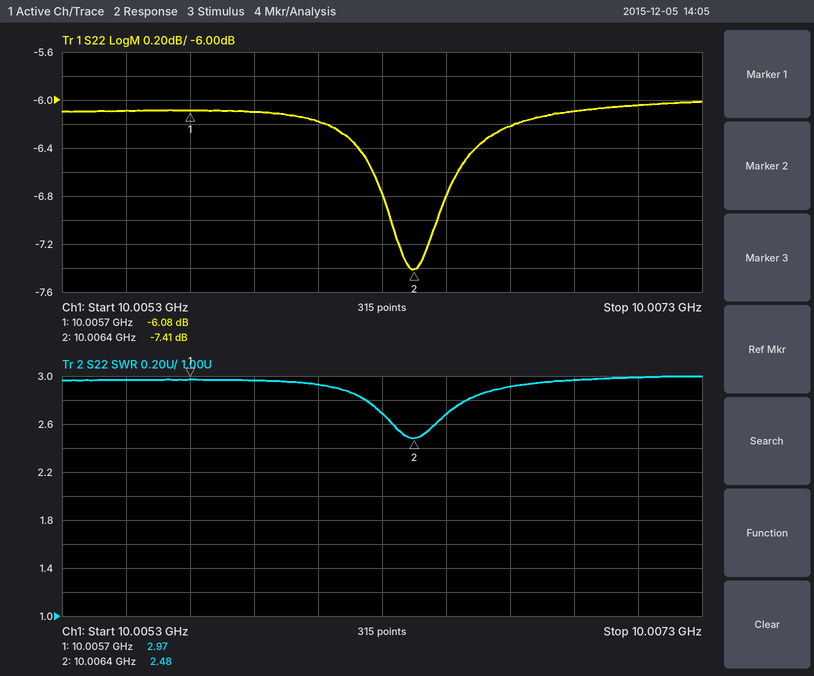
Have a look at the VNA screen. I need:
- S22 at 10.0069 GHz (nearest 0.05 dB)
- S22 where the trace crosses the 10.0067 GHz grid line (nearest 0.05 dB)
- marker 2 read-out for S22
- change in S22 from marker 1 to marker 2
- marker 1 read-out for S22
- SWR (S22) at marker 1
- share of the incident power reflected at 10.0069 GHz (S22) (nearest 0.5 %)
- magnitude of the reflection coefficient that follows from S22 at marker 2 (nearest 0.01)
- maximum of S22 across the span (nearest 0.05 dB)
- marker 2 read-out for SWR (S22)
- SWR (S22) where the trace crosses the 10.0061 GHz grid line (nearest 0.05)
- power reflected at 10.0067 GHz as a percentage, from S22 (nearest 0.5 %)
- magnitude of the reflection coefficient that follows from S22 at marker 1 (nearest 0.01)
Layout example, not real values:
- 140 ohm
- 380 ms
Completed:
- -6.10 dB
- -6.20 dB
- -7.41 dB
- -1.33 dB
- -6.08 dB
- 2.97
- 24.5 %
- 0.43
- -6.00 dB
- 2.48
- 2.95
- 24.0 %
- 0.50
